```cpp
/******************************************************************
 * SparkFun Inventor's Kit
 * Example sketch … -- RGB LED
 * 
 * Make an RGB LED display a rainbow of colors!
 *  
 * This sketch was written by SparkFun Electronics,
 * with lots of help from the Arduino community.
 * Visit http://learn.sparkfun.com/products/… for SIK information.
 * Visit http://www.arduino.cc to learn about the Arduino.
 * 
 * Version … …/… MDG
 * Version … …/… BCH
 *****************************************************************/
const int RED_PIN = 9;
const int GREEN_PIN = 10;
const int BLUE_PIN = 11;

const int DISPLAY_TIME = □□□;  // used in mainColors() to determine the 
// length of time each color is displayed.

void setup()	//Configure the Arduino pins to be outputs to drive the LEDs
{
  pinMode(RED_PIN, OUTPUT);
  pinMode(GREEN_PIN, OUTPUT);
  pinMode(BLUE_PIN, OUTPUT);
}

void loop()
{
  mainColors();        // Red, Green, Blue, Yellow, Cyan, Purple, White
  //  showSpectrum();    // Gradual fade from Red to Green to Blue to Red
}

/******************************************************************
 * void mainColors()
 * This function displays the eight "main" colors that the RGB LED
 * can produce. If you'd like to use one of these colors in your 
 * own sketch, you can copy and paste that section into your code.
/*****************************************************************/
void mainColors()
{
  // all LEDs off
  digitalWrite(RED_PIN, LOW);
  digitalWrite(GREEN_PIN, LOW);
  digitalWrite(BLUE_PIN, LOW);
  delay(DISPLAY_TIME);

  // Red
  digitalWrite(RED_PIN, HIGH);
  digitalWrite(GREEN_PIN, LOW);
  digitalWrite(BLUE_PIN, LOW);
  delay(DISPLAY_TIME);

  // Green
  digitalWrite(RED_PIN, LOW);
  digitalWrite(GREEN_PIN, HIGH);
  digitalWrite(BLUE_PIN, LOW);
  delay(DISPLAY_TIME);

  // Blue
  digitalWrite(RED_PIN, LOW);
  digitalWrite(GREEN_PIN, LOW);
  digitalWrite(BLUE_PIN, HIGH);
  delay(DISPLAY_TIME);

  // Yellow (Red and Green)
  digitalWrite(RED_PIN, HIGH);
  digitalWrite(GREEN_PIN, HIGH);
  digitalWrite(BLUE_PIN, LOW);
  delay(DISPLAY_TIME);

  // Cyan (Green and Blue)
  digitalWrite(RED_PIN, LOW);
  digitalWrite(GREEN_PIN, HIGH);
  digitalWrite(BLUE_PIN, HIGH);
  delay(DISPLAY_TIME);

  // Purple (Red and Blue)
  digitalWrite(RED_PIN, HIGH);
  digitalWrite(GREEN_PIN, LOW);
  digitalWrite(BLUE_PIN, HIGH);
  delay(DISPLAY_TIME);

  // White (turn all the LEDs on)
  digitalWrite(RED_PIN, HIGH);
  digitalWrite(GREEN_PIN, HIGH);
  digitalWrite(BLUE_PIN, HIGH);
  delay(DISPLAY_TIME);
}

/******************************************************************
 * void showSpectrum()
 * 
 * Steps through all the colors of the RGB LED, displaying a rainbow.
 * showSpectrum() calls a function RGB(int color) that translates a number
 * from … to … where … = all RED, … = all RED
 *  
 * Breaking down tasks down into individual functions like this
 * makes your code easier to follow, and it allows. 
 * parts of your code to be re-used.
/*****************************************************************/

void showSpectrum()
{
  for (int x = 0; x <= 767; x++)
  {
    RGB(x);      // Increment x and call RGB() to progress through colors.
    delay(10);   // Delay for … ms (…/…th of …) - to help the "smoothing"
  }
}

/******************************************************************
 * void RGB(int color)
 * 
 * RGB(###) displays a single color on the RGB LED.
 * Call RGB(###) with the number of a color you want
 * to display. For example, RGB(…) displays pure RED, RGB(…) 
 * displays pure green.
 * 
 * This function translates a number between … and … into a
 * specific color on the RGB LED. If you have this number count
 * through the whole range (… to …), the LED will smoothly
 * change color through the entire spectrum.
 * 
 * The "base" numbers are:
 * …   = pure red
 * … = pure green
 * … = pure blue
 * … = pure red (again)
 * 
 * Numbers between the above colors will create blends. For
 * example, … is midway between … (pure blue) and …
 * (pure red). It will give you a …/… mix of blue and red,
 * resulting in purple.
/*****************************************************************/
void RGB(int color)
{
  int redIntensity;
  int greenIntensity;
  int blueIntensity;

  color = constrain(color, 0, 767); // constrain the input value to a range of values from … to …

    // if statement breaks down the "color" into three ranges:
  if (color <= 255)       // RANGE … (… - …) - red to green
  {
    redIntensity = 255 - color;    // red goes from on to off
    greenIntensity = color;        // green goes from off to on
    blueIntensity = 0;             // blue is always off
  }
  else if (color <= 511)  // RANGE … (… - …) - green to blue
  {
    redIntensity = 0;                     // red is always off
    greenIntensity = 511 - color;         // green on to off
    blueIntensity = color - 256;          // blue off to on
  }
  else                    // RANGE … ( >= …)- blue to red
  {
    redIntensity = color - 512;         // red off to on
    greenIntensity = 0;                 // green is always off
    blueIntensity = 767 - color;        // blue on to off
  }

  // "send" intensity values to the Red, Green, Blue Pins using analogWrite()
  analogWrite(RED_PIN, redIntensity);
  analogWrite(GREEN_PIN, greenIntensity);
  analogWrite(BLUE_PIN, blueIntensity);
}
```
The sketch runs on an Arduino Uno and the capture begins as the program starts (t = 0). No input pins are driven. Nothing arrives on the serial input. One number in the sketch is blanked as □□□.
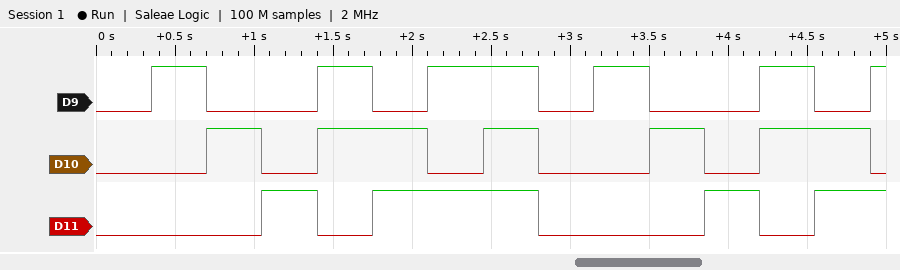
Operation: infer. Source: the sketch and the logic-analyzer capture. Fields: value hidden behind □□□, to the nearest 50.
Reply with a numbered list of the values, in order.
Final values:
1. 350
